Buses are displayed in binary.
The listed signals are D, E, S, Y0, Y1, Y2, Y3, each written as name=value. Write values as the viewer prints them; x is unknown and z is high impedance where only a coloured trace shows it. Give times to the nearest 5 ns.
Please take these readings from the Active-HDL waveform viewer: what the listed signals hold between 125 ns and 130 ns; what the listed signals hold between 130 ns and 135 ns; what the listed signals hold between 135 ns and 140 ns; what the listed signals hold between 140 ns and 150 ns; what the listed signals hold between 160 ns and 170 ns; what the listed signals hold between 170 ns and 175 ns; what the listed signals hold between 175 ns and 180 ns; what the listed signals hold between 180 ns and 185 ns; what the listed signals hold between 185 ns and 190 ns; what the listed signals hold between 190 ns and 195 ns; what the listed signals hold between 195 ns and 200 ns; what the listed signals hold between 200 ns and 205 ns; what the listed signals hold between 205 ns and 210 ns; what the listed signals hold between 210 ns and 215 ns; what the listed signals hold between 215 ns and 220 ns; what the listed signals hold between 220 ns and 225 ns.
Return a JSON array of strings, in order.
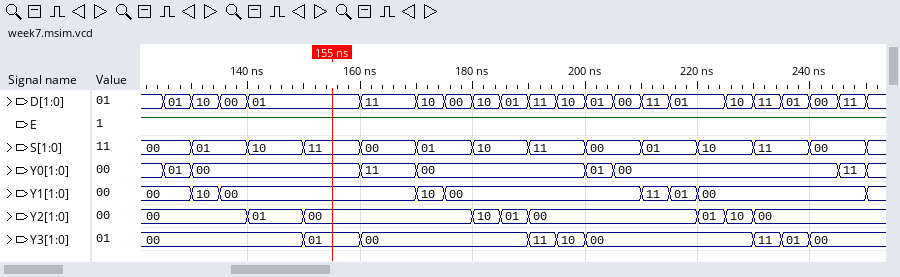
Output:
["D=01, E=1, S=00, Y0=01, Y1=00, Y2=00, Y3=00", "D=10, E=1, S=01, Y0=00, Y1=10, Y2=00, Y3=00", "D=00, E=1, S=01, Y0=00, Y1=00, Y2=00, Y3=00", "D=01, E=1, S=10, Y0=00, Y1=00, Y2=01, Y3=00", "D=11, E=1, S=00, Y0=11, Y1=00, Y2=00, Y3=00", "D=10, E=1, S=01, Y0=00, Y1=10, Y2=00, Y3=00", "D=00, E=1, S=01, Y0=00, Y1=00, Y2=00, Y3=00", "D=10, E=1, S=10, Y0=00, Y1=00, Y2=10, Y3=00", "D=01, E=1, S=10, Y0=00, Y1=00, Y2=01, Y3=00", "D=11, E=1, S=11, Y0=00, Y1=00, Y2=00, Y3=11", "D=10, E=1, S=11, Y0=00, Y1=00, Y2=00, Y3=10", "D=01, E=1, S=00, Y0=01, Y1=00, Y2=00, Y3=00", "D=00, E=1, S=00, Y0=00, Y1=00, Y2=00, Y3=00", "D=11, E=1, S=01, Y0=00, Y1=11, Y2=00, Y3=00", "D=01, E=1, S=01, Y0=00, Y1=01, Y2=00, Y3=00", "D=01, E=1, S=10, Y0=00, Y1=00, Y2=01, Y3=00"]
